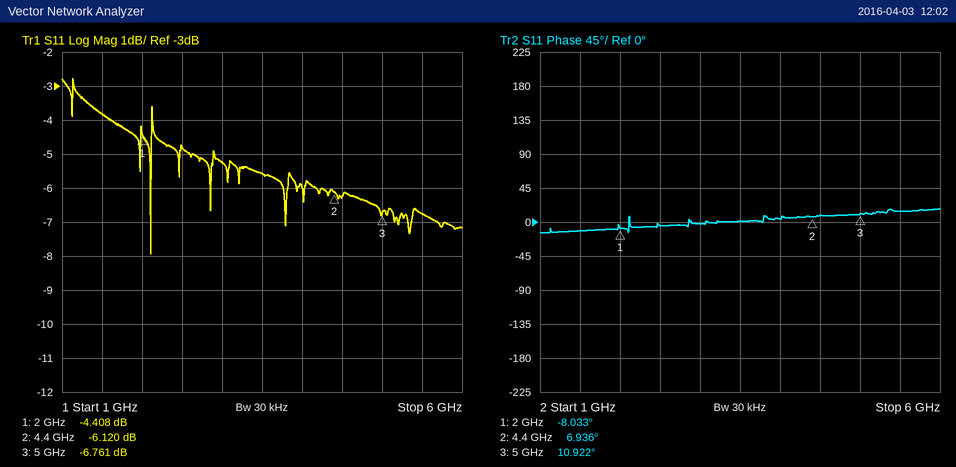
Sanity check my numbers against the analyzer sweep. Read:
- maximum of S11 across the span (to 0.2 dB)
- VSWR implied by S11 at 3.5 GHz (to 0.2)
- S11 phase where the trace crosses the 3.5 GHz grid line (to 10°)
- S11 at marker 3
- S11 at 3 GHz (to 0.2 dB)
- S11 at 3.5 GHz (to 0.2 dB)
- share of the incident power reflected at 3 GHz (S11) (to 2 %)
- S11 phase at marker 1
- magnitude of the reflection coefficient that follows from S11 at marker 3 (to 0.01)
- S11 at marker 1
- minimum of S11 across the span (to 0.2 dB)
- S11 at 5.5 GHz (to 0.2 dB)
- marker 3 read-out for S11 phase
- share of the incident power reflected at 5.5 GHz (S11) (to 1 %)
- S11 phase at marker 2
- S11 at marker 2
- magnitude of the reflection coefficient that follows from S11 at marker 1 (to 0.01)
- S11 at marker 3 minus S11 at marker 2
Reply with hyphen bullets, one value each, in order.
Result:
- -2.8 dB
- 3.2
- 0°
- -6.761 dB
- -5.2 dB
- -5.6 dB
- 30 %
- -8.033°
- 0.46
- -4.408 dB
- -8.0 dB
- -6.8 dB
- 10.922°
- 21 %
- 6.936°
- -6.120 dB
- 0.60
- -0.641 dB
